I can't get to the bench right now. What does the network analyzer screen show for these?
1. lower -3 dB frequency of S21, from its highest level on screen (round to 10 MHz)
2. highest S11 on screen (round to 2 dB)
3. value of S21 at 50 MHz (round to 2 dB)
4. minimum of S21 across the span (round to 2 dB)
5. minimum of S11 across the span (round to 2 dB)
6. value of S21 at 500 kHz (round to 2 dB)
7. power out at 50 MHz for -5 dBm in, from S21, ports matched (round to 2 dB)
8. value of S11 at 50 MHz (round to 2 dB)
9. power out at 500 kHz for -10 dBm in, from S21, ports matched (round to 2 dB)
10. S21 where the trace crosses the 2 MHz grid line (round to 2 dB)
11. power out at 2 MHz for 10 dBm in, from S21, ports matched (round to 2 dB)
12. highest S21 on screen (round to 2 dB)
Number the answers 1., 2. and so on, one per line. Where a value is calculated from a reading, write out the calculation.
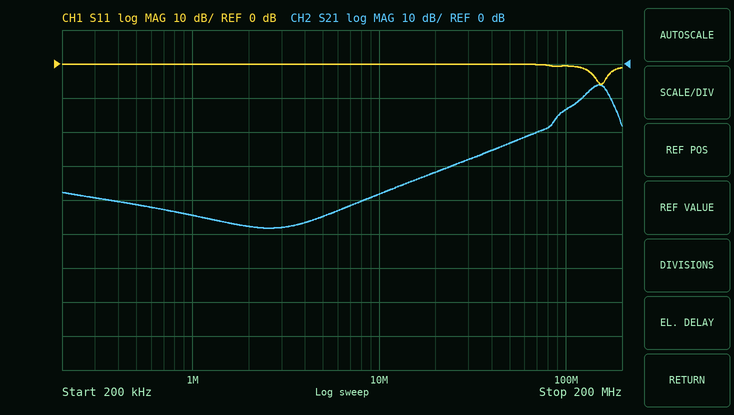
1. 130 MHz
2. 0 dB
3. -24 dB
4. -48 dB
5. -6 dB
6. -42 dB
7. -5 dBm + (-24 dB) = -28 dBm
8. 0 dB
9. -10 dBm + (-42 dB) = -52 dBm
10. -48 dB
11. 10 dBm + (-48 dB) = -38 dBm
12. -6 dB
